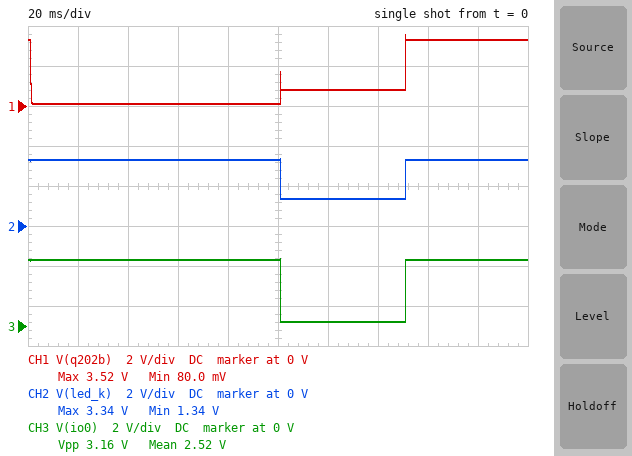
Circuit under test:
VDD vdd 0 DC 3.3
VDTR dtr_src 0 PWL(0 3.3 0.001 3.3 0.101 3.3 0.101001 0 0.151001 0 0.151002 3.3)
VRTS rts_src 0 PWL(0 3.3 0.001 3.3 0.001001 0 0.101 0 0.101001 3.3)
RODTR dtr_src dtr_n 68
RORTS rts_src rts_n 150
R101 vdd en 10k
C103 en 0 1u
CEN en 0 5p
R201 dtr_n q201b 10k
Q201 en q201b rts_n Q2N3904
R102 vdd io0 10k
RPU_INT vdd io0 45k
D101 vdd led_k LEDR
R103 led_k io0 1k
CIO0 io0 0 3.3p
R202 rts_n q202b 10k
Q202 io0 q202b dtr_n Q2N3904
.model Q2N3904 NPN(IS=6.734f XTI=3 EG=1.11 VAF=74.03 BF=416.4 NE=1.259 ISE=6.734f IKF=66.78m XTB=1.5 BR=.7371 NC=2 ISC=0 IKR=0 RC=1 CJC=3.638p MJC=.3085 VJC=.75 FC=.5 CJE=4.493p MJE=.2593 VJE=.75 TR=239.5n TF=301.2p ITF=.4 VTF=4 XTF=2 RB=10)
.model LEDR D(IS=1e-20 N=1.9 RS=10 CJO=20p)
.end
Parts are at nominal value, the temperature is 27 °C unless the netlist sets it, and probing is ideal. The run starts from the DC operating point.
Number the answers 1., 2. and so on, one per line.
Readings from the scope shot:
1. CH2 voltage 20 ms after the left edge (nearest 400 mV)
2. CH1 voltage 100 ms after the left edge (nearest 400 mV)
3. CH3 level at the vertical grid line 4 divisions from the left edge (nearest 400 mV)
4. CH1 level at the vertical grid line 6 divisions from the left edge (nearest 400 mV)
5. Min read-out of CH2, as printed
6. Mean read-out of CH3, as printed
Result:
1. 3.2 V
2. 0 V
3. 3.2 V
4. 800 mV
5. 1.34 V
6. 2.52 V
